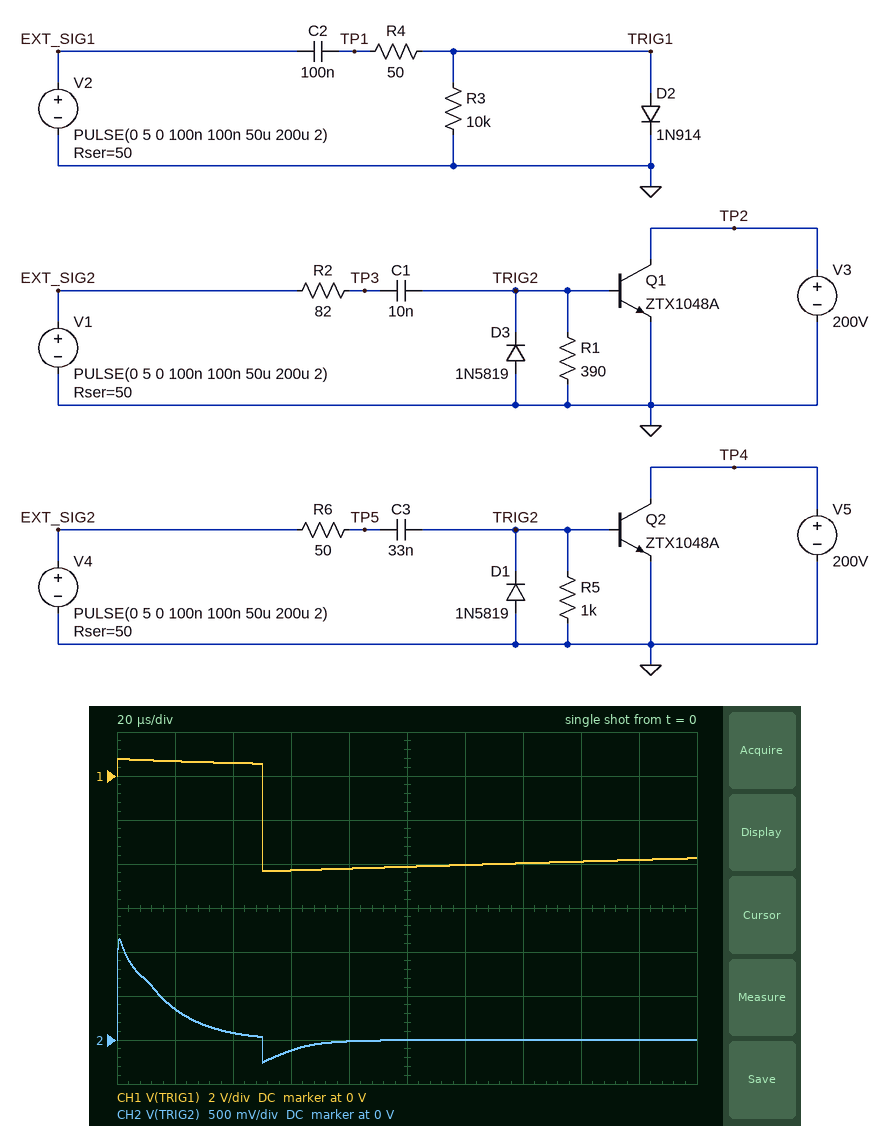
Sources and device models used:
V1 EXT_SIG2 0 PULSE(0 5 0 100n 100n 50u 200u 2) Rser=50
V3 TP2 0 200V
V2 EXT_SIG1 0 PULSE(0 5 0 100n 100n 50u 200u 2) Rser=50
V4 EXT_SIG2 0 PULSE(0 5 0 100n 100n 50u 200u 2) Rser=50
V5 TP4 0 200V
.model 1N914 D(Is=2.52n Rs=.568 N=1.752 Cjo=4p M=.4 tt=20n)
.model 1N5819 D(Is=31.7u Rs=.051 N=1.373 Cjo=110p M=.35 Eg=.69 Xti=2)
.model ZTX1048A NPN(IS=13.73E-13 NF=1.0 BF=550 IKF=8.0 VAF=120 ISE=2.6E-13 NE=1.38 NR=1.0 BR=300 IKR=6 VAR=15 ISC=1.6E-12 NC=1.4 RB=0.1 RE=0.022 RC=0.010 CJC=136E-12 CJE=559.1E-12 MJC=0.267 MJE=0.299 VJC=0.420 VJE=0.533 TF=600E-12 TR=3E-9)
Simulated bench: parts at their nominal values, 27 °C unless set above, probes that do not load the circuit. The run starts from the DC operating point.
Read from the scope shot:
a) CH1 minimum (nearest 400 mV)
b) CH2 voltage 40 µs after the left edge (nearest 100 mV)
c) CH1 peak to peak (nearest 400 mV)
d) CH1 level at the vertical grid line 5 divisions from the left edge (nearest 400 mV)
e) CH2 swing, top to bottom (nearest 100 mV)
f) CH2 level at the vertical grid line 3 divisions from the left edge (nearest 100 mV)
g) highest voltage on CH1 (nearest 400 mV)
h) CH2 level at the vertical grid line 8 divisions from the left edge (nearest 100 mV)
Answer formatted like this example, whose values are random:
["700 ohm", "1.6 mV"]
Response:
["-4.4 V", "100 mV", "5.2 V", "-4.0 V", "1.4 V", "-100 mV", "800 mV", "0 V"]
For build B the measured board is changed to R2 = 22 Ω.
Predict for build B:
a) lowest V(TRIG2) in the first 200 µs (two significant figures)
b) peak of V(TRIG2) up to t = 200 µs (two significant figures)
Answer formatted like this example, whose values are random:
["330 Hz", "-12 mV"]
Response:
["-270 mV", "1.2 V"]
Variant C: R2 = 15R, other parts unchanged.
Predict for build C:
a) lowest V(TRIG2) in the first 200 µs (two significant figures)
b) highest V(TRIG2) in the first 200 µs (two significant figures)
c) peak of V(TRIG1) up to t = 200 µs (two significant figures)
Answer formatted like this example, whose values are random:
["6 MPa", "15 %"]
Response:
["-270 mV", "1.2 V", "780 mV"]
